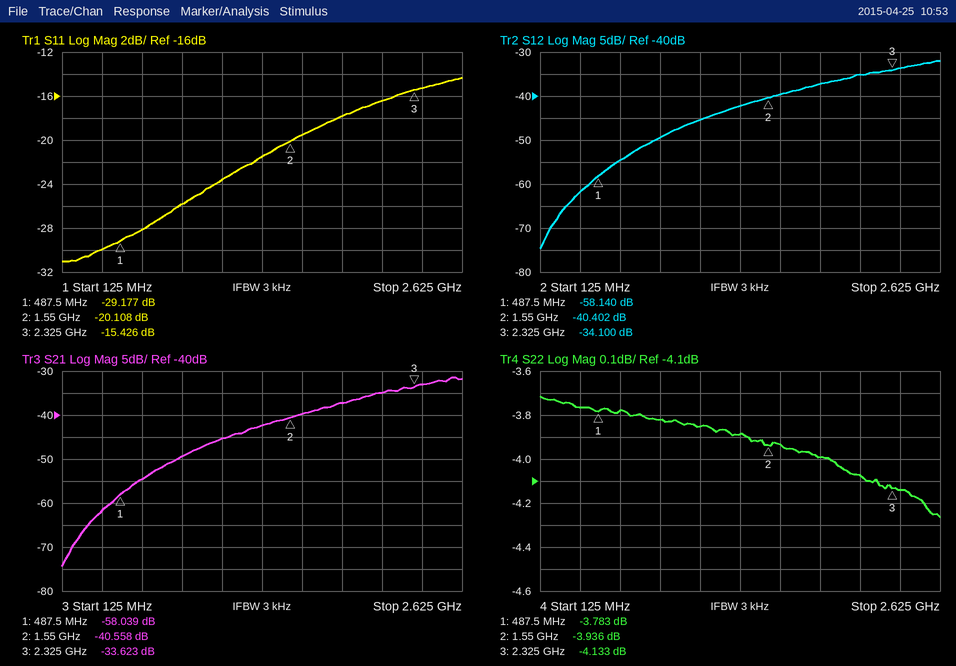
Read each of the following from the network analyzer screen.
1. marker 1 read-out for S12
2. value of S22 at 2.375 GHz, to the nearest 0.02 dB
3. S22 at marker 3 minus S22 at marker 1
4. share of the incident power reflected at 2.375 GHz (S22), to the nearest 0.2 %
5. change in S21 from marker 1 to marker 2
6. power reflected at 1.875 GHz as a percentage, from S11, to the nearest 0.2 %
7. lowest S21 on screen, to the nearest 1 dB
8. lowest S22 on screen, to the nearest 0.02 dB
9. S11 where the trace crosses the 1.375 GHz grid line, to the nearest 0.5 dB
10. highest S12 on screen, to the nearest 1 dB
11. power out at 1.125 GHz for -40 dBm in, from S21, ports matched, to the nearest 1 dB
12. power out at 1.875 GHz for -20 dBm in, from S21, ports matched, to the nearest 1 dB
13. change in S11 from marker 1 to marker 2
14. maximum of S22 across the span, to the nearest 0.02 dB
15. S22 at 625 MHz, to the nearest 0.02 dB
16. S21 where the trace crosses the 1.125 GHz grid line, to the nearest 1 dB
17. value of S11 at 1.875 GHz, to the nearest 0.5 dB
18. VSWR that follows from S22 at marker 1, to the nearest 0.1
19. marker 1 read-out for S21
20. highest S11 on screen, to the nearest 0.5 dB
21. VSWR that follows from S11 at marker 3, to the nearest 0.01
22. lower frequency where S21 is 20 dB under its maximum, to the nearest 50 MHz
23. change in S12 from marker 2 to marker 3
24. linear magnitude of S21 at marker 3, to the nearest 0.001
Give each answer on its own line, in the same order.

-58.140 dB
-4.14 dB
-0.350 dB
38.6 %
17.481 dB
1.6 %
-74 dB
-4.26 dB
-21.5 dB
-32 dB
-85 dBm
-57 dBm
9.069 dB
-3.72 dB
-3.78 dB
-45 dB
-18.0 dB
4.7
-58.039 dB
-14.5 dB
1.41
750 MHz
6.302 dB
0.021
